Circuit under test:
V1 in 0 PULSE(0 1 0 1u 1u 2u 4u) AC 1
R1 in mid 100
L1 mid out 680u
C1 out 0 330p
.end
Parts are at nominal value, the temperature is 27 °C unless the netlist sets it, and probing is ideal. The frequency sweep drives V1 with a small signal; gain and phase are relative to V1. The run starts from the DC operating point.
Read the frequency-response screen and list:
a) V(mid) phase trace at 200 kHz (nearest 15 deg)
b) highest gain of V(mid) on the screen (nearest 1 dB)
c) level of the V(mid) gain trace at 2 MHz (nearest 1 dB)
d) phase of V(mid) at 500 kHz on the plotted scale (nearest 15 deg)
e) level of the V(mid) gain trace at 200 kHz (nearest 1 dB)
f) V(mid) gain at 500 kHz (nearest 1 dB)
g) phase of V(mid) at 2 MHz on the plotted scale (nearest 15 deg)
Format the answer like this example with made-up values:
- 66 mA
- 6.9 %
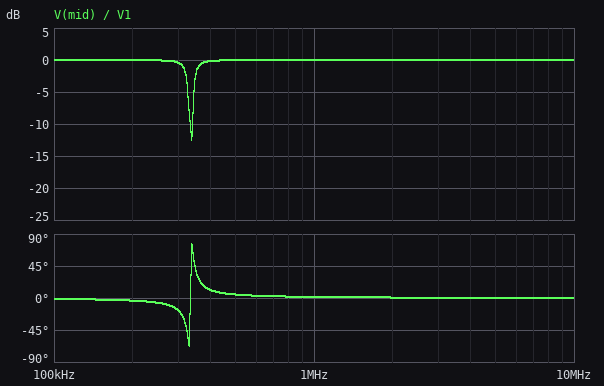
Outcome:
- 0 deg
- 0 dB
- 0 dB
- 0 deg
- 0 dB
- 0 dB
- 0 deg
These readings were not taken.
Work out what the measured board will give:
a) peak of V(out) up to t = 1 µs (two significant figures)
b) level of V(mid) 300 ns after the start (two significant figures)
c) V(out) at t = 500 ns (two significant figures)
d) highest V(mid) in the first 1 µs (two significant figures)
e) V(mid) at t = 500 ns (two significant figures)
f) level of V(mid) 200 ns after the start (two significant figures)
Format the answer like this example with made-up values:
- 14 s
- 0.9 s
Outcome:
- 570 mV
- 290 mV
- 86 mV
- 950 mV
- 480 mV
- 200 mV
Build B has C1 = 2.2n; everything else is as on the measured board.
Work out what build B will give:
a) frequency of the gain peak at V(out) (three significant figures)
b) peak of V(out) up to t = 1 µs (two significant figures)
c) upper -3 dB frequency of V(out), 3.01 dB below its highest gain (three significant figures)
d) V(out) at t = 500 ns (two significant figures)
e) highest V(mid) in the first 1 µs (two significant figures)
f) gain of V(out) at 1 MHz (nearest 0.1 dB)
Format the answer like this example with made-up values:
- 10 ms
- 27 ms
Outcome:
- 129 kHz
- 100 mV
- 140 kHz
- 14 mV
- 930 mV
- -35.3 dB
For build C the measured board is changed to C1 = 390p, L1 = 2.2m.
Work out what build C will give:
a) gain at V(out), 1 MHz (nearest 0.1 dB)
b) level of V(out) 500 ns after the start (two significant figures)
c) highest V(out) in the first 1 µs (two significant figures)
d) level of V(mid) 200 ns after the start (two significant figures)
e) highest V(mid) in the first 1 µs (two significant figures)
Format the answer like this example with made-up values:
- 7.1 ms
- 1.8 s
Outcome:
- -30.3 dB
- 24 mV
- 180 mV
- 200 mV
- 980 mV
